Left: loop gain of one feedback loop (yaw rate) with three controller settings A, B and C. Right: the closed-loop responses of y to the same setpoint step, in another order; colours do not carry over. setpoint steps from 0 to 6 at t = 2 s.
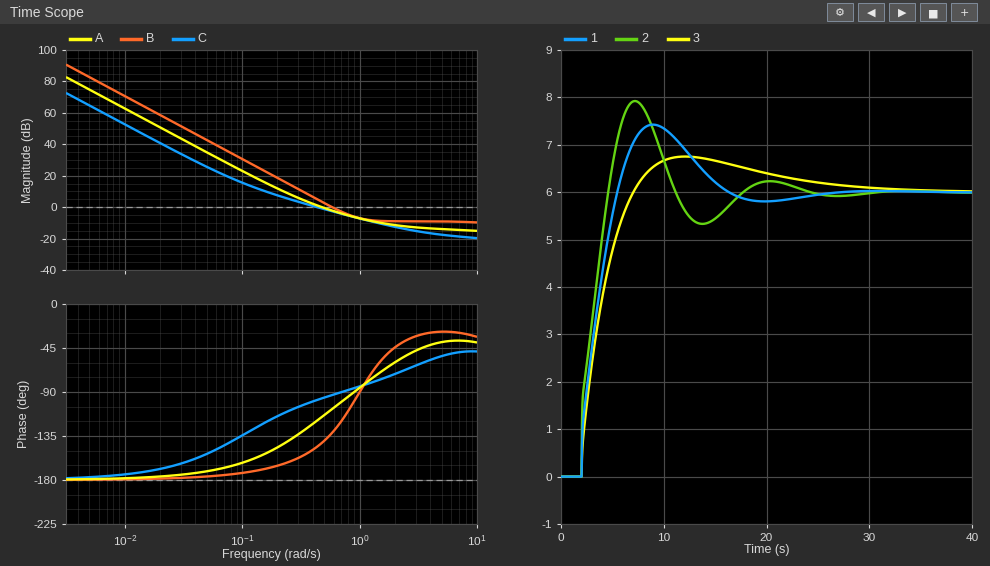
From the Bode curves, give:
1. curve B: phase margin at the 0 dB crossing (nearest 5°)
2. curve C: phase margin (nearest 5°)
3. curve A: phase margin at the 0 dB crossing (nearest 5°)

50°
80°
65°
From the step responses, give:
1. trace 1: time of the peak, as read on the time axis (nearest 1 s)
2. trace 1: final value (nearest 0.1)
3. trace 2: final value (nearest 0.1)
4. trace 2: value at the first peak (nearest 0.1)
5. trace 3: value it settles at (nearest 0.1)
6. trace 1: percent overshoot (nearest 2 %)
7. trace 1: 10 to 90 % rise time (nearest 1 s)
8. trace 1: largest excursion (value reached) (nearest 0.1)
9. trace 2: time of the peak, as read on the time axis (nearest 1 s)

9 s
6.0
6.0
7.9
6.0
24 %
3 s
7.4
7 s
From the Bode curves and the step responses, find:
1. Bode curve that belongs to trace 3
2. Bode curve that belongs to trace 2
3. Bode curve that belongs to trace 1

C
B
A
